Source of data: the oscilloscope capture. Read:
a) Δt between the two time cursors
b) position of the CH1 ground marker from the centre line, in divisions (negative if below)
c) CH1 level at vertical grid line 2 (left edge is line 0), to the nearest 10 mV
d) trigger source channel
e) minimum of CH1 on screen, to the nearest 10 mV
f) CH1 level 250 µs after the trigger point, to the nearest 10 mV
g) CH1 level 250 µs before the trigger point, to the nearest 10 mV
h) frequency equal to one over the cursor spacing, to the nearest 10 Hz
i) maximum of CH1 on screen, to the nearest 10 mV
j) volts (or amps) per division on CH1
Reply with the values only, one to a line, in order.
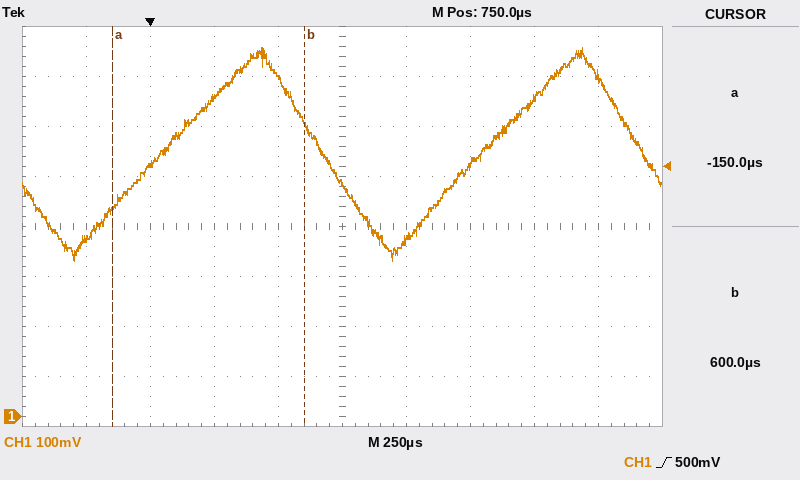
750 µs
-3.8 div
510 mV
CH1
310 mV
640 mV
360 mV
1.33 kHz
740 mV
100 mV
